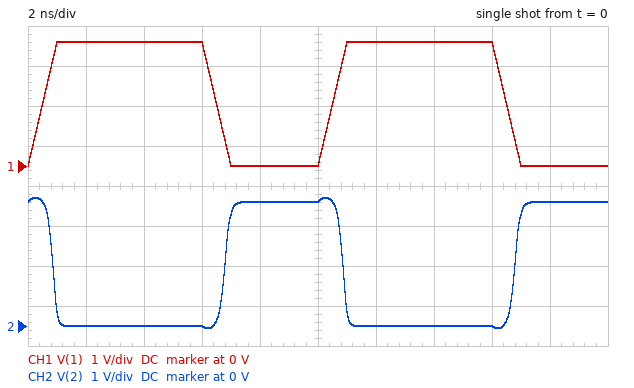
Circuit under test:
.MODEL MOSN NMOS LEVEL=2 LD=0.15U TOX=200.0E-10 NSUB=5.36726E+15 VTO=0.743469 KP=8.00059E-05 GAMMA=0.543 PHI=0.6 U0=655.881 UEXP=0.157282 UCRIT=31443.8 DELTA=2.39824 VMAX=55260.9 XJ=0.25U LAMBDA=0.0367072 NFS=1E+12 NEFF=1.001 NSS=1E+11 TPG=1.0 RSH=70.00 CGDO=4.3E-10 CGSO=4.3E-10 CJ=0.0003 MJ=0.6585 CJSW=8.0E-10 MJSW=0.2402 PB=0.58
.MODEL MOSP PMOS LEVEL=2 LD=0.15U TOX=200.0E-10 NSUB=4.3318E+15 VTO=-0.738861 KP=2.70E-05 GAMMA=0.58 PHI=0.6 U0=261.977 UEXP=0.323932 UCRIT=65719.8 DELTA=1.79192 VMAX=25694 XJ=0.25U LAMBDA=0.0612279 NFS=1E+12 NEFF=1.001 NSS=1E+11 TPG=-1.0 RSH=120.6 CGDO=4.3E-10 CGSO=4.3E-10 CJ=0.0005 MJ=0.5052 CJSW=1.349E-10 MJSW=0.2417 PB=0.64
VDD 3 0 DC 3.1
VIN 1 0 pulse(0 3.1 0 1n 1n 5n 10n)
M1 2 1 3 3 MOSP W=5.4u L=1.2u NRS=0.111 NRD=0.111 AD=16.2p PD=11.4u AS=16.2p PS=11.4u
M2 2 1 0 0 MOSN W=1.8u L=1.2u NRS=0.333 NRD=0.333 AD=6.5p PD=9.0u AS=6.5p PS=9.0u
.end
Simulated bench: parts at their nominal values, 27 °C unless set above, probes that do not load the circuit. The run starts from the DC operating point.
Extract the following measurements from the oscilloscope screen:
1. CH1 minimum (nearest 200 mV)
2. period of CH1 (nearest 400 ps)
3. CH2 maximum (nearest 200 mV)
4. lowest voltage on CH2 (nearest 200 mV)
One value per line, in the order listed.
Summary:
0 V
10.0 ns
3.2 V
0 V
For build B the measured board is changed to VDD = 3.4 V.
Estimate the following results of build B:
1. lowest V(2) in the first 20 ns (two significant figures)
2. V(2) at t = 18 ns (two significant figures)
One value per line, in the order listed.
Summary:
-47 mV
3.4 V
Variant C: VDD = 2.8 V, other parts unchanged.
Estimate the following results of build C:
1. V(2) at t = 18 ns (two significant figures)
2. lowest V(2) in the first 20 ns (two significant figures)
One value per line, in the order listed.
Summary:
2.8 V
-69 mV
